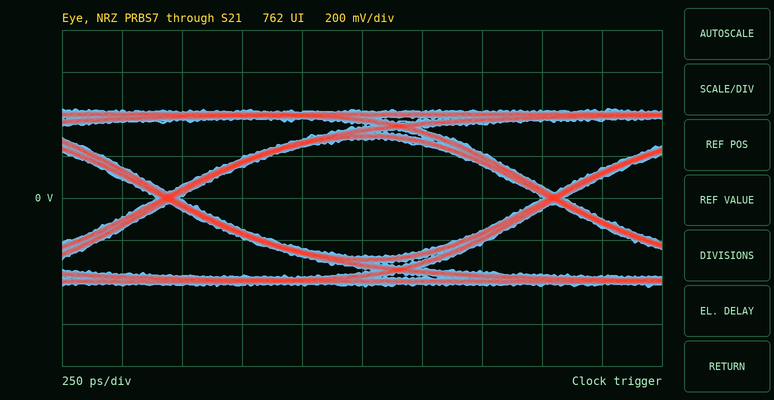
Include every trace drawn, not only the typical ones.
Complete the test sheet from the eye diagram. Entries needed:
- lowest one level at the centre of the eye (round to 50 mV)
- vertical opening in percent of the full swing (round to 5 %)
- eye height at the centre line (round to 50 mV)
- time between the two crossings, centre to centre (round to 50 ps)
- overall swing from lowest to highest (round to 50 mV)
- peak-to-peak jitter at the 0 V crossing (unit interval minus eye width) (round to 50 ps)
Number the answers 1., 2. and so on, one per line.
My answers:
1. 300 mV
2. 65 %
3. 550 mV
4. 1.60 ns
5. 850 mV
6. 100 ps
